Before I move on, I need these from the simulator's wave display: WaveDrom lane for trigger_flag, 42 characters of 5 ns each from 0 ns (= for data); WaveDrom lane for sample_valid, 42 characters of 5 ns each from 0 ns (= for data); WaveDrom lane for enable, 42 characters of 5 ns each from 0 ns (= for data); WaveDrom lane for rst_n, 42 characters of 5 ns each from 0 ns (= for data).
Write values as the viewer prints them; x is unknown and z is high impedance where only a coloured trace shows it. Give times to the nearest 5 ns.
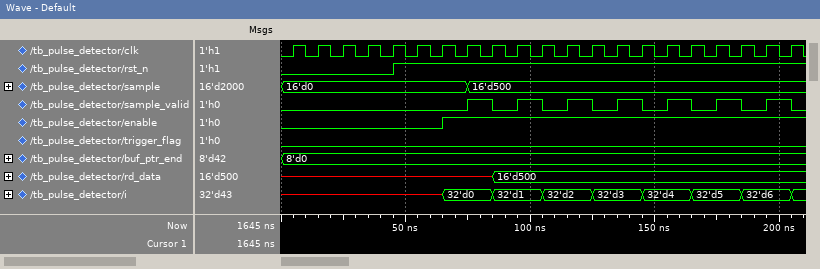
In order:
{name: 'trigger_flag', wave: '0.........................................'}
{name: 'sample_valid', wave: '0..............1.0.1.0.1.0.1.0.1.0.1.0.1.0'}
{name: 'enable', wave: '0............1............................'}
{name: 'rst_n', wave: '0........1................................'}
